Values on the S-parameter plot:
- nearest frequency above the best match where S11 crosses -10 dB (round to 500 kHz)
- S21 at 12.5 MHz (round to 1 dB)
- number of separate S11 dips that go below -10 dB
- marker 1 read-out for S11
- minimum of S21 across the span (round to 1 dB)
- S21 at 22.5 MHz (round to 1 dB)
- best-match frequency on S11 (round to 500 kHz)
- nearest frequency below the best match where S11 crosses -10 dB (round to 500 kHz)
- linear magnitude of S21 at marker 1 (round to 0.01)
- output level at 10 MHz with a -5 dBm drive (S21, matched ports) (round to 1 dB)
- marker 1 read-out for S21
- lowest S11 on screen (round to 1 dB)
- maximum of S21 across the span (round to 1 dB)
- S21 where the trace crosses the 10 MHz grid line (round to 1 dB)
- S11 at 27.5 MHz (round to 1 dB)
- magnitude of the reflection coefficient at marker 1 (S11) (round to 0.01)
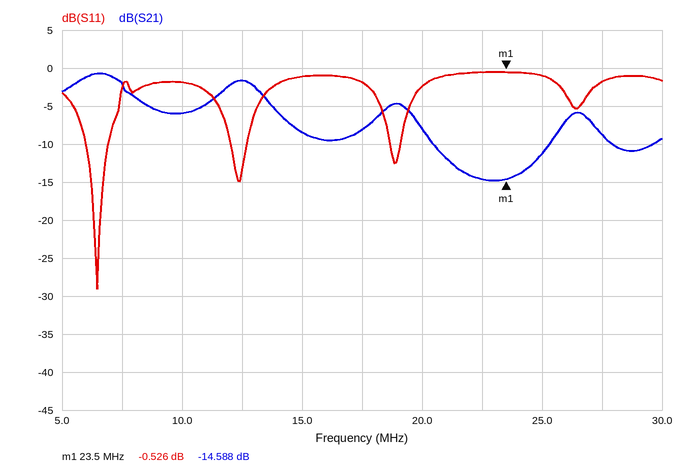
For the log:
7.0 MHz
-2 dB
3
-0.526 dB
-15 dB
-15 dB
6.5 MHz
6.0 MHz
0.19
-11 dBm
-14.588 dB
-29 dB
-1 dB
-6 dB
-2 dB
0.94
